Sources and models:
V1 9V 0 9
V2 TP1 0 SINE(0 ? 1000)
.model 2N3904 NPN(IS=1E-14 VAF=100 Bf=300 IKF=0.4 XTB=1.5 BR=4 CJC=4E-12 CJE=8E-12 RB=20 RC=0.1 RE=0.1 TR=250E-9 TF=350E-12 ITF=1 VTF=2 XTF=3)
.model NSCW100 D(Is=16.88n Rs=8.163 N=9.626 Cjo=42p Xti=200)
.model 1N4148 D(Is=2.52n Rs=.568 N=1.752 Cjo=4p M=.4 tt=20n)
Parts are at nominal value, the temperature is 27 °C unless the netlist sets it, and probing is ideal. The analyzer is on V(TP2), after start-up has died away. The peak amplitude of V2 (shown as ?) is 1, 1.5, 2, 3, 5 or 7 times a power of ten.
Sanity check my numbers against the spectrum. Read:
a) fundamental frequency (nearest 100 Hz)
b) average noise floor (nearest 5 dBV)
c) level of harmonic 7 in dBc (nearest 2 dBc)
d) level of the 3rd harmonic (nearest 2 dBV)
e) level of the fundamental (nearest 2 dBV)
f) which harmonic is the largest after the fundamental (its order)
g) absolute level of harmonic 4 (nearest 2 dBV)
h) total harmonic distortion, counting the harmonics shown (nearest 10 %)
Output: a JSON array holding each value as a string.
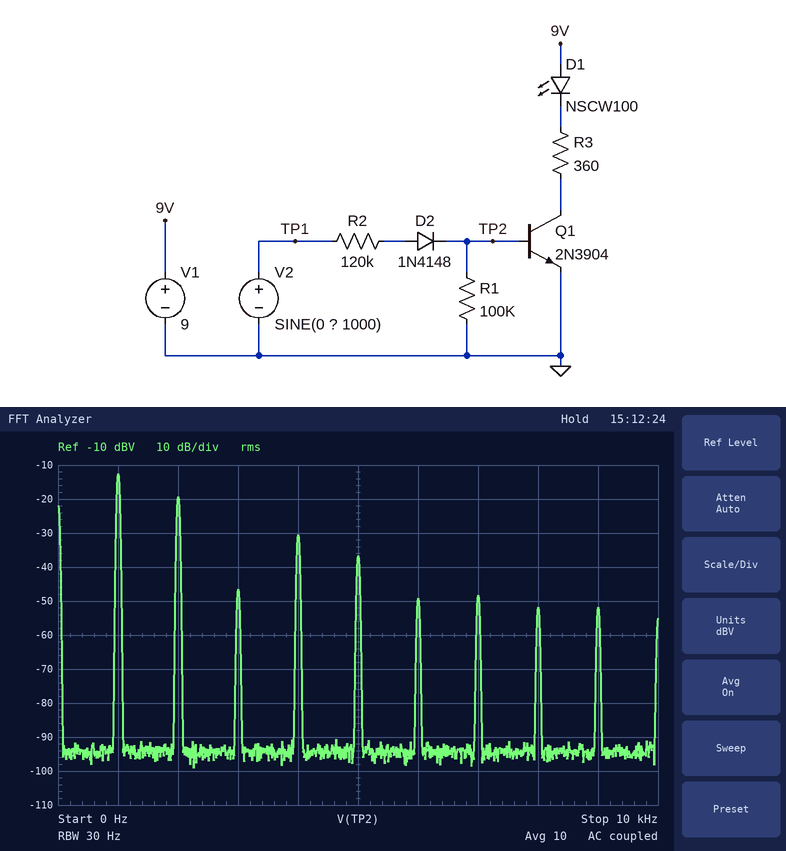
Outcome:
["1.0 kHz", "-95 dBV", "-36 dBc", "-46 dBV", "-12 dBV", "2", "-30 dBV", "50 %"]
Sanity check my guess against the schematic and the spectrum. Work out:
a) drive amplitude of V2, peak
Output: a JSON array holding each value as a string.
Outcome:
["2 V"]
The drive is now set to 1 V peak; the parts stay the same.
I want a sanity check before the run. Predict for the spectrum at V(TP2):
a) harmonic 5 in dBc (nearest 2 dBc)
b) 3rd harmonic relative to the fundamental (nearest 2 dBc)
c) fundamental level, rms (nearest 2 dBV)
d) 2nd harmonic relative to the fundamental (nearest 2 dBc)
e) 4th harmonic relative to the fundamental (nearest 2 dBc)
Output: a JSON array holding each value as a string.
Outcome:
["-26 dBc", "-18 dBc", "-20 dBV", "-6 dBc", "-24 dBc"]
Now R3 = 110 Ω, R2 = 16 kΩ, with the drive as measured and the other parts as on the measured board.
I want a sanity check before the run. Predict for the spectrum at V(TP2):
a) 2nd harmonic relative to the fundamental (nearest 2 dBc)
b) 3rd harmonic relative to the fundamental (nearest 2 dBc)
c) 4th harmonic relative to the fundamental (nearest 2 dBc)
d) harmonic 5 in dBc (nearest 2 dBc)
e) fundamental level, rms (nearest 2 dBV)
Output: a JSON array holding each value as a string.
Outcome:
["-8 dBc", "-18 dBc", "-14 dBc", "-28 dBc", "-10 dBV"]
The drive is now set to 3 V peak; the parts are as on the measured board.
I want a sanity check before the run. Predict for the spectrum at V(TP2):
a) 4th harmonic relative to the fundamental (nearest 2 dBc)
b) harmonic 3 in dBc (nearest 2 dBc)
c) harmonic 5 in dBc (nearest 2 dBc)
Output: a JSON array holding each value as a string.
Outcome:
["-14 dBc", "-18 dBc", "-32 dBc"]
